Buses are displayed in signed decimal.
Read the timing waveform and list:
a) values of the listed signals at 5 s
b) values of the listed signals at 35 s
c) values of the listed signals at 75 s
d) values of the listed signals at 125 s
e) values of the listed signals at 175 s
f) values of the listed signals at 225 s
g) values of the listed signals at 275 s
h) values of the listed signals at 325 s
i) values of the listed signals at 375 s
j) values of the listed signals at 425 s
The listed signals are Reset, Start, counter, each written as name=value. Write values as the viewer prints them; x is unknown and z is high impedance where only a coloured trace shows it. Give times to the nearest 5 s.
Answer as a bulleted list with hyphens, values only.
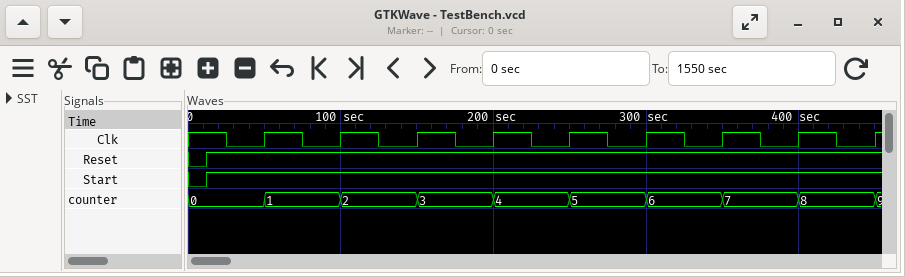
- Reset=0, Start=0, counter=0
- Reset=1, Start=1, counter=0
- Reset=1, Start=1, counter=1
- Reset=1, Start=1, counter=2
- Reset=1, Start=1, counter=3
- Reset=1, Start=1, counter=4
- Reset=1, Start=1, counter=5
- Reset=1, Start=1, counter=6
- Reset=1, Start=1, counter=7
- Reset=1, Start=1, counter=8
